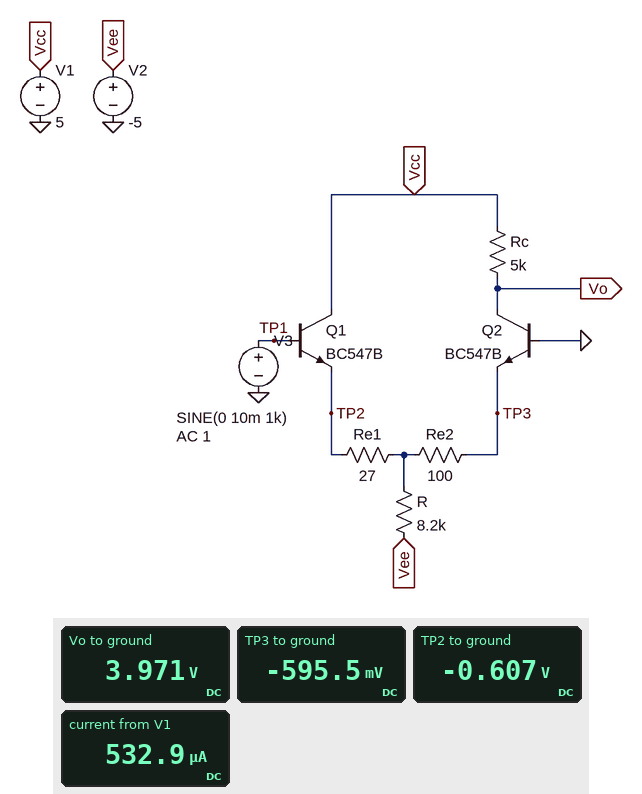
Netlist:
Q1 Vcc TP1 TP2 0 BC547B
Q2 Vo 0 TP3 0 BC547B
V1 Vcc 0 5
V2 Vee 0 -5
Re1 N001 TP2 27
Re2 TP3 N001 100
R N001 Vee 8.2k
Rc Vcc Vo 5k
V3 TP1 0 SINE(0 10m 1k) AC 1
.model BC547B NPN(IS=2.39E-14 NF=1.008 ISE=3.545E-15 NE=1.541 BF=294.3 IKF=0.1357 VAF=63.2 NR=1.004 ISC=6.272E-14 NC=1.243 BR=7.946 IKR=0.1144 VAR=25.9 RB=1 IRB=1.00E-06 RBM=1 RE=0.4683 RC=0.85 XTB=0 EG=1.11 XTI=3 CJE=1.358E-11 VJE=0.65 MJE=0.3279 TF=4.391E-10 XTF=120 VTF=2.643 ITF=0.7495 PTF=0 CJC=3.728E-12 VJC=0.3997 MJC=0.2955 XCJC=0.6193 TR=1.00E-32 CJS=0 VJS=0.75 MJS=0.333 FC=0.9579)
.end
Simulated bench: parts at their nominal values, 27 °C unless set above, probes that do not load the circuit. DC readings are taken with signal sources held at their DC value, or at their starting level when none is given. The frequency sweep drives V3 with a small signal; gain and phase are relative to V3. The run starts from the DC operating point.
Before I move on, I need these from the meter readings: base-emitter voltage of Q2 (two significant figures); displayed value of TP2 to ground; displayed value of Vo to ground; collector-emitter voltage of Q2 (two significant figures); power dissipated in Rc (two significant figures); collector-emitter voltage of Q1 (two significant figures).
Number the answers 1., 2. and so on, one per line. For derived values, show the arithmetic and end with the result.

1. 0 V - (-595.5 mV) = 600 mV
2. -0.607 V
3. 3.971 V
4. 3.971 V - (-595.5 mV) = 4.6 V
5. (5 V - 3.971 V)^2 / 5 kΩ = 210 µW
6. 5 V - (-607 mV) = 5.6 V
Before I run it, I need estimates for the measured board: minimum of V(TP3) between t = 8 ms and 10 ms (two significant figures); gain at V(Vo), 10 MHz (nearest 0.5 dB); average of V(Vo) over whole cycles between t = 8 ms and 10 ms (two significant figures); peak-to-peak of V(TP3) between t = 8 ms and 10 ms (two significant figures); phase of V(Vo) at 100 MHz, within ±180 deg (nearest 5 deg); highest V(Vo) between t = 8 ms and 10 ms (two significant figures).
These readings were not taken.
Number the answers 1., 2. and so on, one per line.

1. -600 mV
2. 22.0 dB
3. 4.0 V
4. 7.6 mV
5. -125 deg
6. 4.1 V
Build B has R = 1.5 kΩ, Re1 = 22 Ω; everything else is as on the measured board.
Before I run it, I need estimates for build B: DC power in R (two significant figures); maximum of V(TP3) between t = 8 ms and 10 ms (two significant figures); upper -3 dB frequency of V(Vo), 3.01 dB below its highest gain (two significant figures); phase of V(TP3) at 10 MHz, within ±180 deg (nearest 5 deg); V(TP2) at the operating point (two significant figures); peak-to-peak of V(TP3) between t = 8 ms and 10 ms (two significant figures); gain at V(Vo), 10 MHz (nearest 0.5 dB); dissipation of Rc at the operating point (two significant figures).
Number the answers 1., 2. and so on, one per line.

1. 12 mW
2. -630 mV
3. 13 MHz
4. -5 deg
5. -660 mV
6. 4.3 mV
7. 27.0 dB
8. 2.7 mW
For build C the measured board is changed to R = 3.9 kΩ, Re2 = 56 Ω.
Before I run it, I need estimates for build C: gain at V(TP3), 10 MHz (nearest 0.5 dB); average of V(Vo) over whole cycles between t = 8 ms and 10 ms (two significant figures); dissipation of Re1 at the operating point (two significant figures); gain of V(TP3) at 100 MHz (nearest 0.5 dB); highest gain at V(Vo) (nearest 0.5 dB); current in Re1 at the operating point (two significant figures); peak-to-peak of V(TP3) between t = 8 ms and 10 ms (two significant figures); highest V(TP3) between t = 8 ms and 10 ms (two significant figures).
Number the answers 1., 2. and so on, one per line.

1. -10.0 dB
2. 2.7 V
3. 12 µW
4. -12.0 dB
5. 28.5 dB
6. 650 µA
7. 6.4 mV
8. -610 mV
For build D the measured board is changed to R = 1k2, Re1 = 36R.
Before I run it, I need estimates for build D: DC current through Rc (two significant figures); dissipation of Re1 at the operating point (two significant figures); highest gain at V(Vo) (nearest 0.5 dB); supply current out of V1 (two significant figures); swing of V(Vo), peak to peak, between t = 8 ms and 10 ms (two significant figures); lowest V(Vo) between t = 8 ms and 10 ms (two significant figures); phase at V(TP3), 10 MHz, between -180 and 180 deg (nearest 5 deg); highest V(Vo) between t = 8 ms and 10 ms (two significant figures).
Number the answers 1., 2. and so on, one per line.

1. 1.1 mA
2. 220 µW
3. 29.0 dB
4. 3.5 mA
5. 440 mV
6. -570 mV
7. -5 deg
8. -130 mV
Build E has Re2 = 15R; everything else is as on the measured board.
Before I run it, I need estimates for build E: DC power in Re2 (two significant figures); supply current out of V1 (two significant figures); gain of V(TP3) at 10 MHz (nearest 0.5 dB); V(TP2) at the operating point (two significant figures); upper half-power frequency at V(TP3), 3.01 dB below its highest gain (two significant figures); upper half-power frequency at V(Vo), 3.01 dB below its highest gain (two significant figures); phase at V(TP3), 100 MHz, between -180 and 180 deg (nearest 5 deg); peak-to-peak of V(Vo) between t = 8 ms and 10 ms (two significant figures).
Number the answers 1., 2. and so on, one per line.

1. 1.2 µW
2. 530 µA
3. -8.0 dB
4. -600 mV
5. 250 MHz
6. 17 MHz
7. -20 deg
8. 410 mV
